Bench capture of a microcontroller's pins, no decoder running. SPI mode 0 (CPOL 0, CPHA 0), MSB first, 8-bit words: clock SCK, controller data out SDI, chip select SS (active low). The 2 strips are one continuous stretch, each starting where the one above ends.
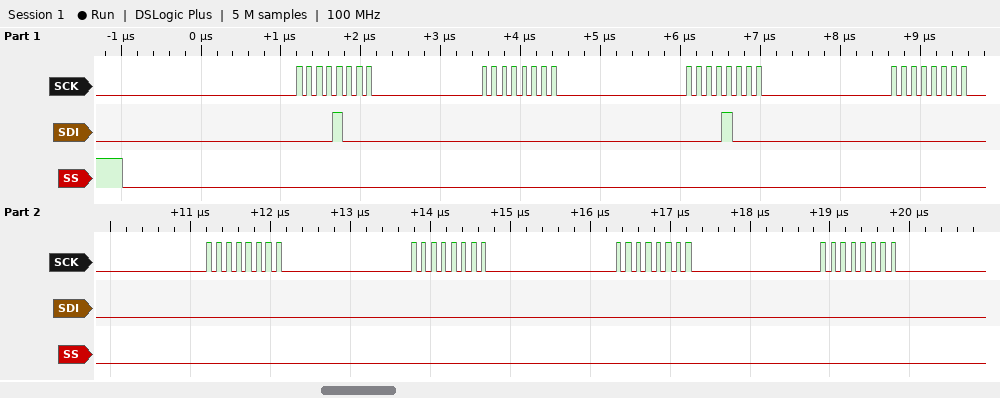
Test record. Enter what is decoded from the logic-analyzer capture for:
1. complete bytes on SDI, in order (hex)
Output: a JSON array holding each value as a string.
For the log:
["08 00 08 00 00 00 00 00"]
